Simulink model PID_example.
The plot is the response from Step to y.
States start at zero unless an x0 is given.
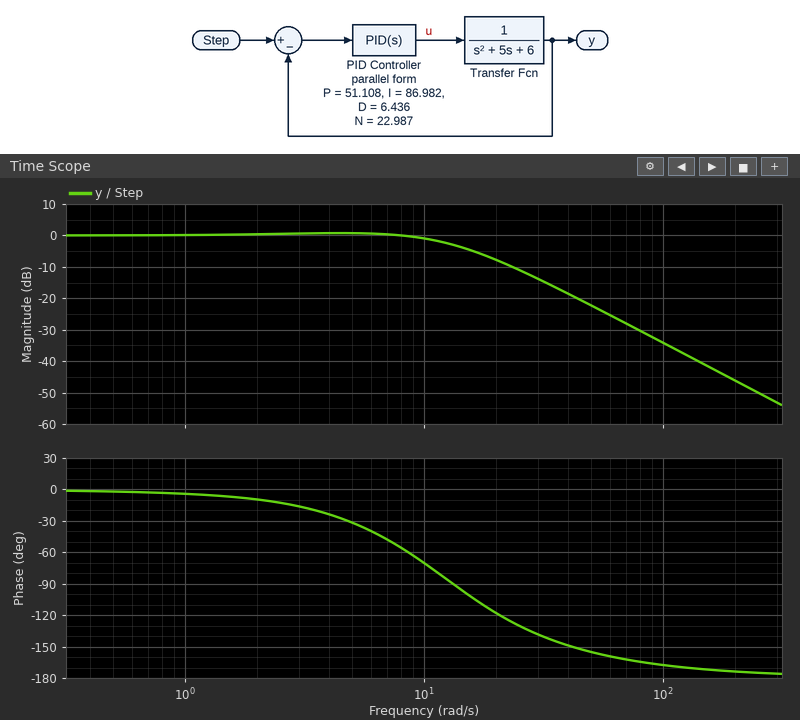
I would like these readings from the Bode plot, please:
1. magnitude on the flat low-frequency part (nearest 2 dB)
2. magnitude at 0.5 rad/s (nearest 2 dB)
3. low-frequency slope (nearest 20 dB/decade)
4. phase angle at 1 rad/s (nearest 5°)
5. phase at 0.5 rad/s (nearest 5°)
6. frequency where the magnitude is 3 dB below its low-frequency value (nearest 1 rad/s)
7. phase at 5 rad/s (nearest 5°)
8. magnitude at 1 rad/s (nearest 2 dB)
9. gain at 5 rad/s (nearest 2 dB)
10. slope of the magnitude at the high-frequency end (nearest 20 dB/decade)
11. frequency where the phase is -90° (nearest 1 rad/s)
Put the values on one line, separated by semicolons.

0 dB; 0 dB; 0 dB/decade; -5°; 0°; 13 rad/s; -30°; 0 dB; 0 dB; -40 dB/decade; 13 rad/s
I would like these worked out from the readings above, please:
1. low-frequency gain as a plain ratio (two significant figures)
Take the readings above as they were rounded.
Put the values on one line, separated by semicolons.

1.0
